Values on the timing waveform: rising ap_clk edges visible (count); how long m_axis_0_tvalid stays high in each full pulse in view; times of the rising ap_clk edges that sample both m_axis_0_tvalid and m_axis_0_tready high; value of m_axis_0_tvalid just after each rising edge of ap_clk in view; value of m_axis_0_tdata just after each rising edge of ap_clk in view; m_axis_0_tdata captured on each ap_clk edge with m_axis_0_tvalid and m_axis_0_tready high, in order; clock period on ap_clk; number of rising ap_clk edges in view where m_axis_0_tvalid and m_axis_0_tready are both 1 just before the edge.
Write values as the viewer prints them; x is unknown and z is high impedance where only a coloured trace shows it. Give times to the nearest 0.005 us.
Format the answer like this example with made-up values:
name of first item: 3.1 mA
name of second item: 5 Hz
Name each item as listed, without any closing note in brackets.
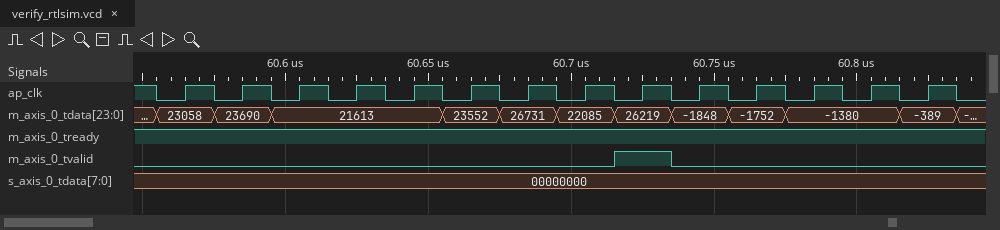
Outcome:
rising ap_clk edges visible: 14
how long m_axis_0_tvalid stays high in each full pulse in view: 0.02 us
times of the rising ap_clk edges that sample both m_axis_0_tvalid and m_axis_0_tready high: 60.725 us
value of m_axis_0_tvalid just after each rising edge of ap_clk in view: 0 0 0 0 0 0 0 0 1 0 0 0 0 0
value of m_axis_0_tdata just after each rising edge of ap_clk in view: 23058, 23690, 21613, 21613, 21613, 23552, 26731, 22085, 26219, -1848, -1752, -1380, -1380, -389
m_axis_0_tdata captured on each ap_clk edge with m_axis_0_tvalid and m_axis_0_tready high, in order: 26219
clock period on ap_clk: 0.02 us
number of rising ap_clk edges in view where m_axis_0_tvalid and m_axis_0_tready are both 1 just before the edge: 1
